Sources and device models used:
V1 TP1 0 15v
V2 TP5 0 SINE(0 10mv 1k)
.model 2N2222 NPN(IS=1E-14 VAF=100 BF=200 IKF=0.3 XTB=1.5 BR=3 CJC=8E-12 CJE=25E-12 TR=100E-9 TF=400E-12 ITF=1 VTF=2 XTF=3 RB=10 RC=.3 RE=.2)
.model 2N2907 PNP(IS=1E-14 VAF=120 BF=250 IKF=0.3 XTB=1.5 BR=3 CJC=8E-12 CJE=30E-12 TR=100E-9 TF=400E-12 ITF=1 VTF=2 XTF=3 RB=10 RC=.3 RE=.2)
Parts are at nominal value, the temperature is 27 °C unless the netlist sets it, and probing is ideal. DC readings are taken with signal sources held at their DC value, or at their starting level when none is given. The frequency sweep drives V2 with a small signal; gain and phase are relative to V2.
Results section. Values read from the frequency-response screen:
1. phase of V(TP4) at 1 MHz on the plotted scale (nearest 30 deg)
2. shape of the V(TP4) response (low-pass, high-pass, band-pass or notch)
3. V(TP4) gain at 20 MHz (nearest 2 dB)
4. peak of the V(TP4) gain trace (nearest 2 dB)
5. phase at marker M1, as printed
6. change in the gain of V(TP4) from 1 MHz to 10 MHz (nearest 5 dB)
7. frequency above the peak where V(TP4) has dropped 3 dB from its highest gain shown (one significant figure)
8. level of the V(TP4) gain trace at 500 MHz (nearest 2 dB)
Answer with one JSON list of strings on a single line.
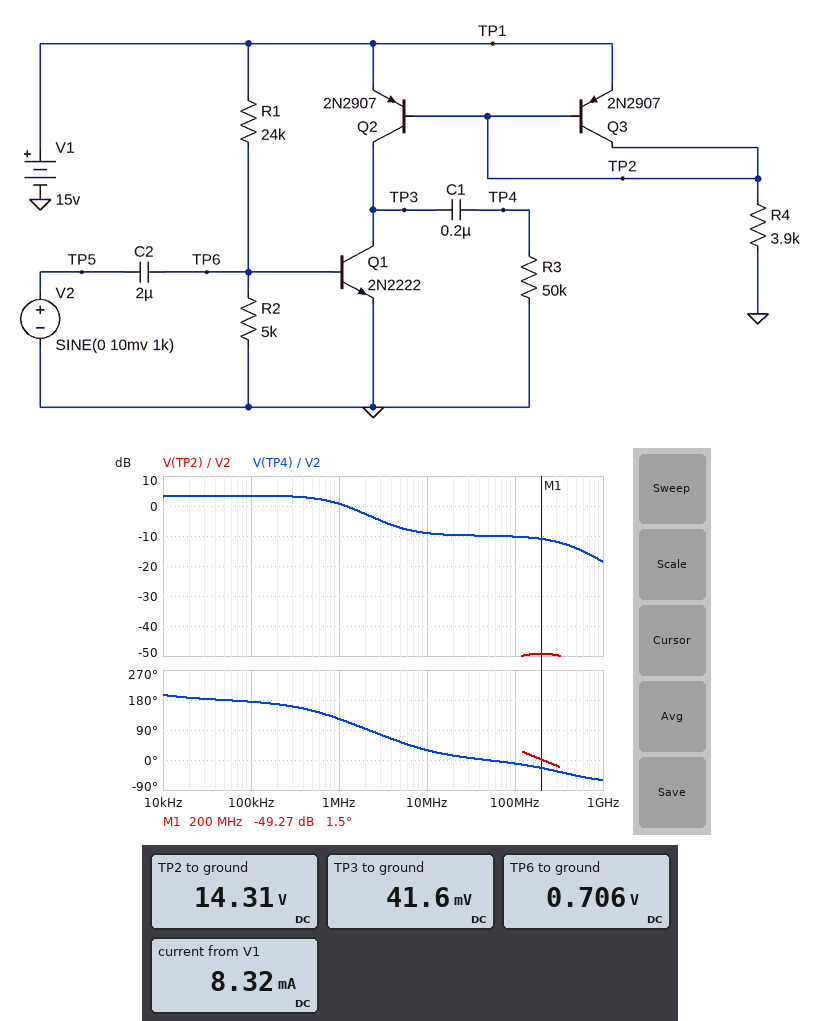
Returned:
["120 deg", "low-pass", "-10 dB", "4 dB", "1.5 deg", "-10 dB", "1 MHz", "-14 dB"]
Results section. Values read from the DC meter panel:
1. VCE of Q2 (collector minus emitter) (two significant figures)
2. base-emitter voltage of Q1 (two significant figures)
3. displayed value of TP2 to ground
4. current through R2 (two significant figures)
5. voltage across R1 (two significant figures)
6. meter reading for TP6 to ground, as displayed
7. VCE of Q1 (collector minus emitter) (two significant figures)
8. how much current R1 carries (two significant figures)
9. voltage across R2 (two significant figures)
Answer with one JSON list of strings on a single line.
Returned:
["-15 V", "710 mV", "14.31 V", "140 µA", "14 V", "0.706 V", "42 mV", "600 µA", "710 mV"]
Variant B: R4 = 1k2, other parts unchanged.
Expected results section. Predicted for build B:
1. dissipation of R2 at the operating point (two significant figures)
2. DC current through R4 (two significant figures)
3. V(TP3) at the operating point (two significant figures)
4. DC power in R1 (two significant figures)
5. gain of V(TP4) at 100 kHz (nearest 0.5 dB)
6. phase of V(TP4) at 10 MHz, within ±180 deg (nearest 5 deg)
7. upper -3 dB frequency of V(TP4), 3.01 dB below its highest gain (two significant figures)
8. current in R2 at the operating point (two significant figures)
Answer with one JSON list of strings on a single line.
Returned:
["110 µW", "12 mA", "74 mV", "8.5 mW", "11.0 dB", "60 deg", "780 kHz", "150 µA"]
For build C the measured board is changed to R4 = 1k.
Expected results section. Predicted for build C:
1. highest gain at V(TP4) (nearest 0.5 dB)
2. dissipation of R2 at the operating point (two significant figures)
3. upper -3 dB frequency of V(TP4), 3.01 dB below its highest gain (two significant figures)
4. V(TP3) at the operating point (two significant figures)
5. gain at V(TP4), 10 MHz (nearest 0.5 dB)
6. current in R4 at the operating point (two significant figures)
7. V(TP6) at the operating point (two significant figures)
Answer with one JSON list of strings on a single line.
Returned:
["12.0 dB", "110 µW", "750 kHz", "81 mV", "-9.5 dB", "14 mA", "740 mV"]
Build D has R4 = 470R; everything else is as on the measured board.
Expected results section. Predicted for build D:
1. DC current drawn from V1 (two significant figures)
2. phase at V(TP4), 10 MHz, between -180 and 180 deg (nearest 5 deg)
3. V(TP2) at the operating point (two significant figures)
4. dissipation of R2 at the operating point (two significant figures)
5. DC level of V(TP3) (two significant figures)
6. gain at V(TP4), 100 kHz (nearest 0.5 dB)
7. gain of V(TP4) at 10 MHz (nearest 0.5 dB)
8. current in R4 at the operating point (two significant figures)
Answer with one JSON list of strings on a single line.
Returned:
["64 mA", "80 deg", "14 V", "120 µW", "120 mV", "17.0 dB", "-6.5 dB", "30 mA"]
